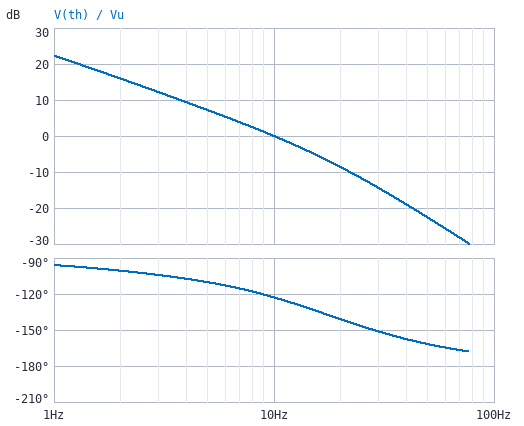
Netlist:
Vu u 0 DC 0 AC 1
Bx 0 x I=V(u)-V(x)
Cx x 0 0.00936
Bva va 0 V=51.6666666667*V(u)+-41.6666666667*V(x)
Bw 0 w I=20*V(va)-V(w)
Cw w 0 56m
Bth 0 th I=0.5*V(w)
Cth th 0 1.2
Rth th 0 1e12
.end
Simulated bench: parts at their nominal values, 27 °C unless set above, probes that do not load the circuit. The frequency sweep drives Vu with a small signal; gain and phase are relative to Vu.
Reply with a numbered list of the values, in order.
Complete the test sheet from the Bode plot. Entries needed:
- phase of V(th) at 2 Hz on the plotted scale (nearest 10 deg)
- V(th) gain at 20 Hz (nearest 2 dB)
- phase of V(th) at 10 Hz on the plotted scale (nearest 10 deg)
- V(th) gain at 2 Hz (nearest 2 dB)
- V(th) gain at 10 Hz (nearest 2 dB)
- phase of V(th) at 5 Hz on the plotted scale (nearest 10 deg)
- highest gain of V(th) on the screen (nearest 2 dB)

1. -100 deg
2. -8 dB
3. -120 deg
4. 16 dB
5. 0 dB
6. -110 deg
7. 22 dB
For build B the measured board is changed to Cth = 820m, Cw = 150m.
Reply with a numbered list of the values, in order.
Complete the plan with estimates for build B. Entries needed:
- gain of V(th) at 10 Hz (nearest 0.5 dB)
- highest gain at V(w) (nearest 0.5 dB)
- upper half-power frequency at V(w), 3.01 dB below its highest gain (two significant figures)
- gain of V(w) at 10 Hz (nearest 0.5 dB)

1. -5.0 dB
2. 46.0 dB
3. 1.2 Hz
4. 35.5 dB
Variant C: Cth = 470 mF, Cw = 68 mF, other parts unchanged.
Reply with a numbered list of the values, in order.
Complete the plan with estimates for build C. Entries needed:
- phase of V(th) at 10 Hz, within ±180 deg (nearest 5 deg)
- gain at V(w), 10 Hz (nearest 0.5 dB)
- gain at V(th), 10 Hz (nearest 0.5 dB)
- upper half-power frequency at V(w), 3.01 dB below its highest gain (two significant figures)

1. -125 deg
2. 42.0 dB
3. 6.5 dB
4. 6.2 Hz
